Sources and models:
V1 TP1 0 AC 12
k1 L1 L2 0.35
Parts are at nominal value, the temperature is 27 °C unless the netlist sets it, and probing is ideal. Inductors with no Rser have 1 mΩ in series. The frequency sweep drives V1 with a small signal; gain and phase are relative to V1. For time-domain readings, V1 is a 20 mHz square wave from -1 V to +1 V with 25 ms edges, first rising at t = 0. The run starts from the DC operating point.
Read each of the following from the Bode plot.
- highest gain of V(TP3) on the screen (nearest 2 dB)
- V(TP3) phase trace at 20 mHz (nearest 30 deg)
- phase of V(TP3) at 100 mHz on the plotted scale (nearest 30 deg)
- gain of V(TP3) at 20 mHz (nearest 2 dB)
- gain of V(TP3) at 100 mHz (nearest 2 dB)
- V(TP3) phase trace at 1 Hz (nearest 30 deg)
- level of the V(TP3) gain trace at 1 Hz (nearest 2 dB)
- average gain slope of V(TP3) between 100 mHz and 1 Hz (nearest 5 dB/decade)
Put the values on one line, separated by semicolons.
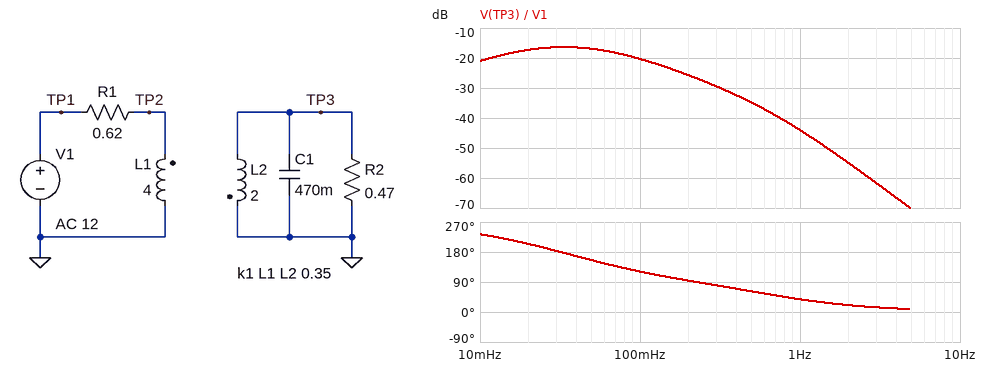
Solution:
-16 dB; 210 deg; 120 deg; -18 dB; -20 dB; 30 deg; -44 dB; -25 dB/decade
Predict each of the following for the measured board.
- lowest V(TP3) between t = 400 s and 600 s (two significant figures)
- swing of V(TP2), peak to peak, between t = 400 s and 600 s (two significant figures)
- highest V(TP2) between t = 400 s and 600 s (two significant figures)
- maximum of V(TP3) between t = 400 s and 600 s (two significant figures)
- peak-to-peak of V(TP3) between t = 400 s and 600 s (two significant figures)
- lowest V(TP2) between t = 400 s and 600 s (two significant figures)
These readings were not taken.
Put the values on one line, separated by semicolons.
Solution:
-220 mV; 3.9 V; 1.9 V; 220 mV; 440 mV; -1.9 V
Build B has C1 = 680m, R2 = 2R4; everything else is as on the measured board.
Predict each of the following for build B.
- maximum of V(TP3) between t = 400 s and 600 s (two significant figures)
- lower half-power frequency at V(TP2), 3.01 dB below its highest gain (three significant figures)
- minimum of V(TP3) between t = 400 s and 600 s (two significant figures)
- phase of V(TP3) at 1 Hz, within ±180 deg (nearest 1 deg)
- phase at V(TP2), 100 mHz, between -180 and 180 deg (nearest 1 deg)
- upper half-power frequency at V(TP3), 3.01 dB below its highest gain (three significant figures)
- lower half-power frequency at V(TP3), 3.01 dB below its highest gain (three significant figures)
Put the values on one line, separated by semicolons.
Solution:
490 mV; 25.1 mHz; -490 mV; 7 deg; 13 deg; 175 mHz; 62.5 mHz
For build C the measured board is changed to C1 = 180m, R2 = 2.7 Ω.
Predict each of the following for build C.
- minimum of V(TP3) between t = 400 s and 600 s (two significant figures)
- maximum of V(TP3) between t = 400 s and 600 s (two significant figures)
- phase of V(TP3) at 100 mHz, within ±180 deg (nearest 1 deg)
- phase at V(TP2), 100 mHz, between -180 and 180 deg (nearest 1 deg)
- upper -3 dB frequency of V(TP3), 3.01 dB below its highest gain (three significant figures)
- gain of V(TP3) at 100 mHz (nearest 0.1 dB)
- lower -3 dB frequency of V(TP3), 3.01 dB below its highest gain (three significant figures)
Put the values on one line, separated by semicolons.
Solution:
-450 mV; 450 mV; 169 deg; 14 deg; 323 mHz; -12.2 dB; 26.6 mHz
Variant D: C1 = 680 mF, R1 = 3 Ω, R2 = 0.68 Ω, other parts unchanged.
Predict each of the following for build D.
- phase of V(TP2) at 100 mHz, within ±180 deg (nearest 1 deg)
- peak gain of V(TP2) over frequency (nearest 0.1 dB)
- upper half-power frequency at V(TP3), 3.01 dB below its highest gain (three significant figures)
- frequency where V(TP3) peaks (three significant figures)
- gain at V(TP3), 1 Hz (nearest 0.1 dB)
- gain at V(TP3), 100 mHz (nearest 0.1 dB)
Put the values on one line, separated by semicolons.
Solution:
51 deg; 0 dB; 199 mHz; 87.5 mHz; -46.0 dB; -21.5 dB
